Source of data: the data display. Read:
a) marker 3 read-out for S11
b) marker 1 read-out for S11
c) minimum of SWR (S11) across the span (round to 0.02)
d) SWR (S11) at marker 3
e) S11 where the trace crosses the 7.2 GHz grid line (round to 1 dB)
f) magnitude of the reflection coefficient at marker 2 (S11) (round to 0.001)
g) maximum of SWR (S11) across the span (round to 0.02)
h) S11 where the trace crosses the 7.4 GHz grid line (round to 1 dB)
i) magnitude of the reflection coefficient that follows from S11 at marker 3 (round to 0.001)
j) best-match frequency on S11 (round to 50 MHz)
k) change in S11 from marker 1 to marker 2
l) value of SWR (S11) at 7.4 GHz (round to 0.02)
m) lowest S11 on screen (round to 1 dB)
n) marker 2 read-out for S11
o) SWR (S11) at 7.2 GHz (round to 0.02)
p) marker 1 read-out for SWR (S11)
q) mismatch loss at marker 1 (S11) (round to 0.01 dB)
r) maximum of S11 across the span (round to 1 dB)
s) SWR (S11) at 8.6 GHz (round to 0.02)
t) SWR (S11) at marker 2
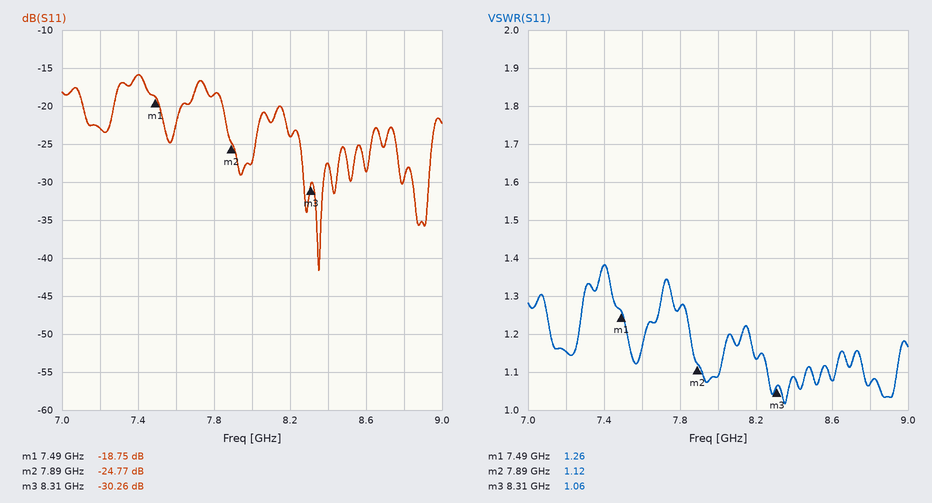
-30.26 dB
-18.75 dB
1.02
1.06
-23 dB
0.058
1.38
-16 dB
0.031
8.35 GHz
-6.02 dB
1.38
-42 dB
-24.77 dB
1.16
1.26
0.06 dB
-16 dB
1.08
1.12
